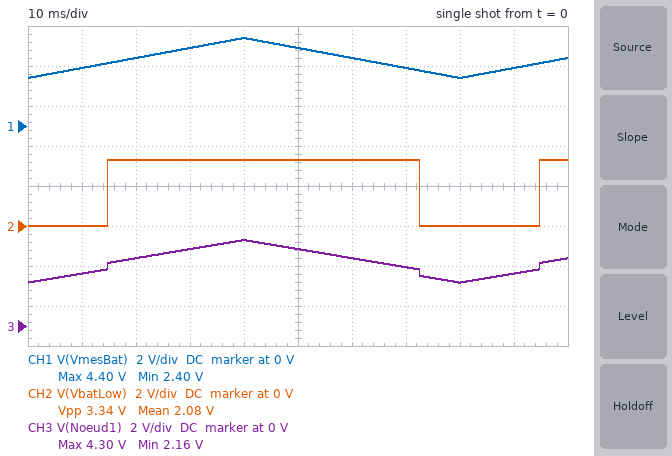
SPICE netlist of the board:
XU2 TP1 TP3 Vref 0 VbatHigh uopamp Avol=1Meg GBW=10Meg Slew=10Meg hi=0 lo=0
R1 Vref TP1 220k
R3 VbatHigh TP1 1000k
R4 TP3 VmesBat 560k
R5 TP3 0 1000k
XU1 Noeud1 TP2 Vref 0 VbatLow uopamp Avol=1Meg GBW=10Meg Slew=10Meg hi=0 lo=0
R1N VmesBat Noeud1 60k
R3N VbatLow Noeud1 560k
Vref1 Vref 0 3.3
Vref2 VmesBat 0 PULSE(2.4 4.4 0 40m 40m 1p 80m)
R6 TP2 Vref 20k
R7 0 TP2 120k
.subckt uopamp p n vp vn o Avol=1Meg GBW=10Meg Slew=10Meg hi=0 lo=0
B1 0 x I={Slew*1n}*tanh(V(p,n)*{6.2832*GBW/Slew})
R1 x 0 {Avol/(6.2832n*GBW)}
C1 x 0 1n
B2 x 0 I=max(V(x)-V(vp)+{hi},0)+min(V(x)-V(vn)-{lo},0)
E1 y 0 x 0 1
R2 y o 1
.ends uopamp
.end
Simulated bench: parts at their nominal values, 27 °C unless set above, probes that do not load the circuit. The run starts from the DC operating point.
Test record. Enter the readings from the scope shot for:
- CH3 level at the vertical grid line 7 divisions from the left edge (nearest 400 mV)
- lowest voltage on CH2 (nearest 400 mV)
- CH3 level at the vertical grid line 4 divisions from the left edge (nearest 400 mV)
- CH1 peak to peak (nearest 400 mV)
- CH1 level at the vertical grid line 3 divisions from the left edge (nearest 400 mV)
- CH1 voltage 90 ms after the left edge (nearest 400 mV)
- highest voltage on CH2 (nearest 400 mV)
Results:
2.8 V
0 V
4.4 V
2.0 V
4.0 V
2.8 V
3.2 V
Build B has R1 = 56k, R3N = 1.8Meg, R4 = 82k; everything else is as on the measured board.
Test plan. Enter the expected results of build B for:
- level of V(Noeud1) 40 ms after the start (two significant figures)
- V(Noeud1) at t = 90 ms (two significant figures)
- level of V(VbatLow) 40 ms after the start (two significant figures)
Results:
4.4 V
2.8 V
3.3 V
